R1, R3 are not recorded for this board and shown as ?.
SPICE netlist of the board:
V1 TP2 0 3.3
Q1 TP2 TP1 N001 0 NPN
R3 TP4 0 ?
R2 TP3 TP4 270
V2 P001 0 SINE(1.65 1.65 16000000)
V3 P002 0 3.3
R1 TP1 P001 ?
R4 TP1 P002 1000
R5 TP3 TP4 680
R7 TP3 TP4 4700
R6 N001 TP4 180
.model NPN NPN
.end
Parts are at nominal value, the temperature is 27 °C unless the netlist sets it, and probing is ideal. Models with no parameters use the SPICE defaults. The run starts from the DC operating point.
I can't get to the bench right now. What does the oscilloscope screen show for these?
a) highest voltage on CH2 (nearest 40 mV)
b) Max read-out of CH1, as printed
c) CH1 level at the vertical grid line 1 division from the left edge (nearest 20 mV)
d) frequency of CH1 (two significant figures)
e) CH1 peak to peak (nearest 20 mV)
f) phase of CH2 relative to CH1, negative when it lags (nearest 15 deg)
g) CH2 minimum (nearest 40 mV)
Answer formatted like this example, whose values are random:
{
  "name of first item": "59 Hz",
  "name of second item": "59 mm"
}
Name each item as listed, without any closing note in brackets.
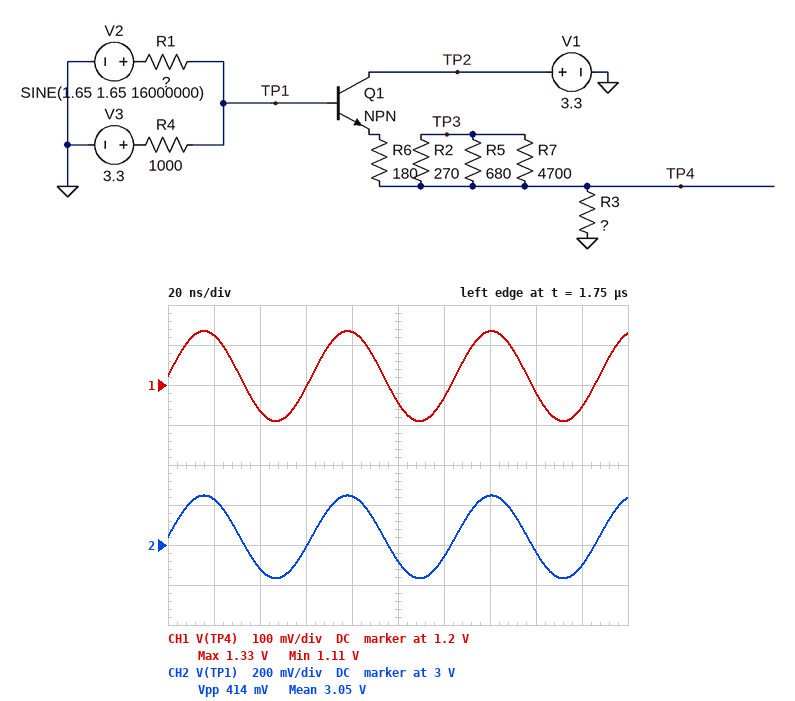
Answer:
{
  "highest voltage on CH2": "3.24 V",
  "Max read-out of CH1, as printed": "1.33 V",
  "CH1 level at the vertical grid line 1 division from the left edge": "1.32 V",
  "frequency of CH1": "16 MHz",
  "CH1 peak to peak": "220 mV",
  "phase of CH2 relative to CH1, negative when it lags": "0 deg",
  "CH2 minimum": "2.84 V"
}
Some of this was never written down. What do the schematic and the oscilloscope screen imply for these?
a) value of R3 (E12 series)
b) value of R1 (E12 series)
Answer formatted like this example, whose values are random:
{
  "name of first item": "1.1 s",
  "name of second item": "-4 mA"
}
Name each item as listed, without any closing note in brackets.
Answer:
{
  "value of R3": "220 Ω",
  "value of R1": "6.8 kΩ"
}
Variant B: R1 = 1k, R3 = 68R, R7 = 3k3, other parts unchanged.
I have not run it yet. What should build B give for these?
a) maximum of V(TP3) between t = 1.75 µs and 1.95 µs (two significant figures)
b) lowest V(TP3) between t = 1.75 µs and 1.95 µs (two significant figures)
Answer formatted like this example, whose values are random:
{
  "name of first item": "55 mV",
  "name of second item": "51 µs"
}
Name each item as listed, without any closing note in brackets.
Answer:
{
  "maximum of V(TP3) between t = 1.75 µs and 1.95 µs": "660 mV",
  "lowest V(TP3) between t = 1.75 µs and 1.95 µs": "230 mV"
}
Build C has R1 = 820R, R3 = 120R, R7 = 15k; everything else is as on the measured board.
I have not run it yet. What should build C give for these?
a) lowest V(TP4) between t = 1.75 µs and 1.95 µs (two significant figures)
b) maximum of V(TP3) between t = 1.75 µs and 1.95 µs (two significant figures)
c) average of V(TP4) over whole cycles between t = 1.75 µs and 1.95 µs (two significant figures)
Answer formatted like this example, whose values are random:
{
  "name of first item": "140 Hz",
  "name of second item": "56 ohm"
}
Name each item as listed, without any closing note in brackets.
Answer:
{
  "lowest V(TP4) between t = 1.75 µs and 1.95 µs": "270 mV",
  "maximum of V(TP3) between t = 1.75 µs and 1.95 µs": "970 mV",
  "average of V(TP4) over whole cycles between t = 1.75 µs and 1.95 µs": "620 mV"
}
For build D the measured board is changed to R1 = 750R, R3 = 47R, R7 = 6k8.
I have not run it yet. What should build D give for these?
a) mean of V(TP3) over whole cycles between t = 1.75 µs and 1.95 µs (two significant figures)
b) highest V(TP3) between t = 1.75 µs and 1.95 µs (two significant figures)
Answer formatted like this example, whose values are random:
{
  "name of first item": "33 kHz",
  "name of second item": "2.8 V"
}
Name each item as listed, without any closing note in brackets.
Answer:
{
  "mean of V(TP3) over whole cycles between t = 1.75 µs and 1.95 µs": "310 mV",
  "highest V(TP3) between t = 1.75 µs and 1.95 µs": "500 mV"
}
